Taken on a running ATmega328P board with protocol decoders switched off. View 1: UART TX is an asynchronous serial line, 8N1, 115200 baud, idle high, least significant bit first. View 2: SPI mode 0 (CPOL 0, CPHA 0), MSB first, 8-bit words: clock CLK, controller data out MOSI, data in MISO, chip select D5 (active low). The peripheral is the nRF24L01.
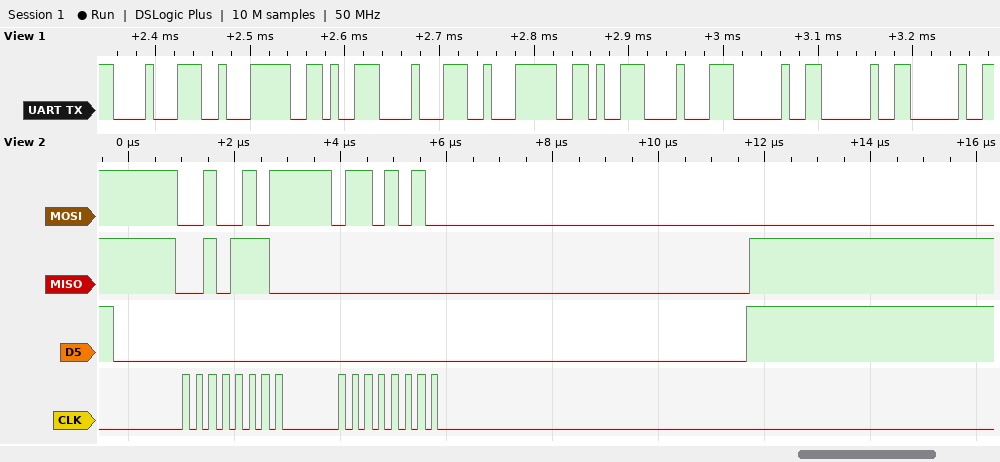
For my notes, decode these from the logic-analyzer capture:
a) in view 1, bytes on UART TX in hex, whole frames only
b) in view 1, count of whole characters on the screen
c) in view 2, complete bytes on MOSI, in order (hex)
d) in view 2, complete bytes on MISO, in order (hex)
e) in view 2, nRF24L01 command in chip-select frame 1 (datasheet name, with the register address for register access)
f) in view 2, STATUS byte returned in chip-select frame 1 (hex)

0x88 0xE2 0x96 0x88 0xE2 0x96 0x88 0x20 0x20 0x20
10
25 6A
2E 00
W_REGISTER 0x05
0x2E
